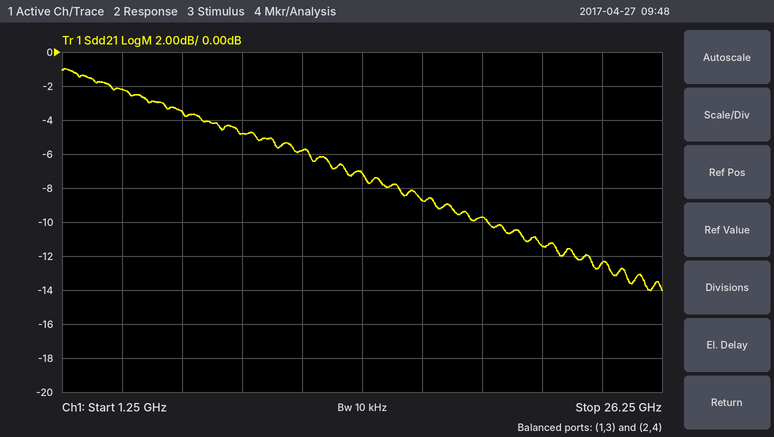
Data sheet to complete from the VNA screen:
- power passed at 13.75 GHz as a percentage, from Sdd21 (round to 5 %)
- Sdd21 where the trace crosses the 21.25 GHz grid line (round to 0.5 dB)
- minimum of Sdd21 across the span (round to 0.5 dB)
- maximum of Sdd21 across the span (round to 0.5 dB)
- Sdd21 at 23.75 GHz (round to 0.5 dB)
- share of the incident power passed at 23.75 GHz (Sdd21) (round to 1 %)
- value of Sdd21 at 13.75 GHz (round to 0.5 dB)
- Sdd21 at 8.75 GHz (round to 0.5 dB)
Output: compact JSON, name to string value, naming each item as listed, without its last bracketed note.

{"power passed at 13.75 GHz as a percentage, from Sdd21": "20 %", "Sdd21 where the trace crosses the 21.25 GHz grid line": "-11.5 dB", "minimum of Sdd21 across the span": "-14.0 dB", "maximum of Sdd21 across the span": "-1.0 dB", "Sdd21 at 23.75 GHz": "-12.5 dB", "share of the incident power passed at 23.75 GHz (Sdd21)": "6 %", "value of Sdd21 at 13.75 GHz": "-7.0 dB", "Sdd21 at 8.75 GHz": "-5.0 dB"}
